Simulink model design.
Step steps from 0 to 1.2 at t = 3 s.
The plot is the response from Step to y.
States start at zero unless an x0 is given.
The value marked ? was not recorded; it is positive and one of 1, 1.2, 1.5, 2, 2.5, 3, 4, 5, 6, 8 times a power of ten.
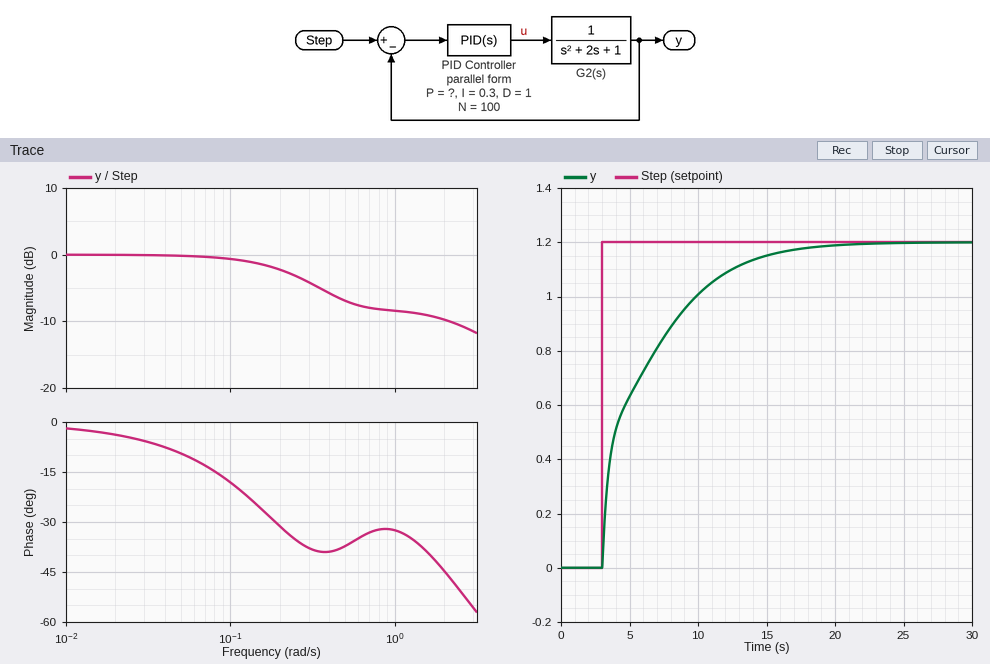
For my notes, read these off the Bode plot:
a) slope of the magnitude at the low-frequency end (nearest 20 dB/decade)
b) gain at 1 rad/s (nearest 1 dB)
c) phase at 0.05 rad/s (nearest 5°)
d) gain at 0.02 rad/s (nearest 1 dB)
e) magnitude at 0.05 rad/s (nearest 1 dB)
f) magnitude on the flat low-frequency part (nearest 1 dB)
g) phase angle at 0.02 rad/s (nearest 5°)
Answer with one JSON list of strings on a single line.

["0 dB/decade", "-8 dB", "-10°", "0 dB", "0 dB", "0 dB", "-5°"]
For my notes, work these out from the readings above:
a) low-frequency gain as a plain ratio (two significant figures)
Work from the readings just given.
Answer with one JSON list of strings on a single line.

["1.0"]
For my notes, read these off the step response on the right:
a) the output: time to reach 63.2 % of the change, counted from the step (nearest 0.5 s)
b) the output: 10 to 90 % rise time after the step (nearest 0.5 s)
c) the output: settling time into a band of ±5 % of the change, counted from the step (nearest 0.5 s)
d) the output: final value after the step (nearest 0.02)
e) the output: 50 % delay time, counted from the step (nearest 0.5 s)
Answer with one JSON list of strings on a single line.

["3.5 s", "8.5 s", "11.5 s", "1.20", "1.5 s"]
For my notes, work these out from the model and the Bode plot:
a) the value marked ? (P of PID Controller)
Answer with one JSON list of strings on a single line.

["0.8"]
